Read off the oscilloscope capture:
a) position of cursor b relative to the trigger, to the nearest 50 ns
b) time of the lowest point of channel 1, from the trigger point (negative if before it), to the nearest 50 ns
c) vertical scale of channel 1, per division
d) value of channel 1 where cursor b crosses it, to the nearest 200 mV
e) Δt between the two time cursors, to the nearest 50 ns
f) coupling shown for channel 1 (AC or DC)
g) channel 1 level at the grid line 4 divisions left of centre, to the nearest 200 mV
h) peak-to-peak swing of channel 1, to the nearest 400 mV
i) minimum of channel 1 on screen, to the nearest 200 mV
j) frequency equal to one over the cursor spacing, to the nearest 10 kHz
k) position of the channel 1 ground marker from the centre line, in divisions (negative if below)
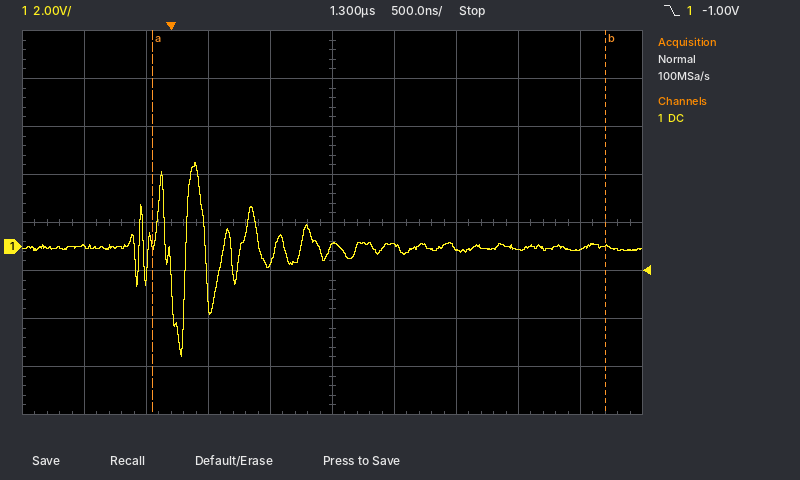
+3.50 µs
+100 ns
2 V
0.0 V
3.65 µs
DC
0.0 V
8.0 V
-4.6 V
270 kHz
-0.5 div
